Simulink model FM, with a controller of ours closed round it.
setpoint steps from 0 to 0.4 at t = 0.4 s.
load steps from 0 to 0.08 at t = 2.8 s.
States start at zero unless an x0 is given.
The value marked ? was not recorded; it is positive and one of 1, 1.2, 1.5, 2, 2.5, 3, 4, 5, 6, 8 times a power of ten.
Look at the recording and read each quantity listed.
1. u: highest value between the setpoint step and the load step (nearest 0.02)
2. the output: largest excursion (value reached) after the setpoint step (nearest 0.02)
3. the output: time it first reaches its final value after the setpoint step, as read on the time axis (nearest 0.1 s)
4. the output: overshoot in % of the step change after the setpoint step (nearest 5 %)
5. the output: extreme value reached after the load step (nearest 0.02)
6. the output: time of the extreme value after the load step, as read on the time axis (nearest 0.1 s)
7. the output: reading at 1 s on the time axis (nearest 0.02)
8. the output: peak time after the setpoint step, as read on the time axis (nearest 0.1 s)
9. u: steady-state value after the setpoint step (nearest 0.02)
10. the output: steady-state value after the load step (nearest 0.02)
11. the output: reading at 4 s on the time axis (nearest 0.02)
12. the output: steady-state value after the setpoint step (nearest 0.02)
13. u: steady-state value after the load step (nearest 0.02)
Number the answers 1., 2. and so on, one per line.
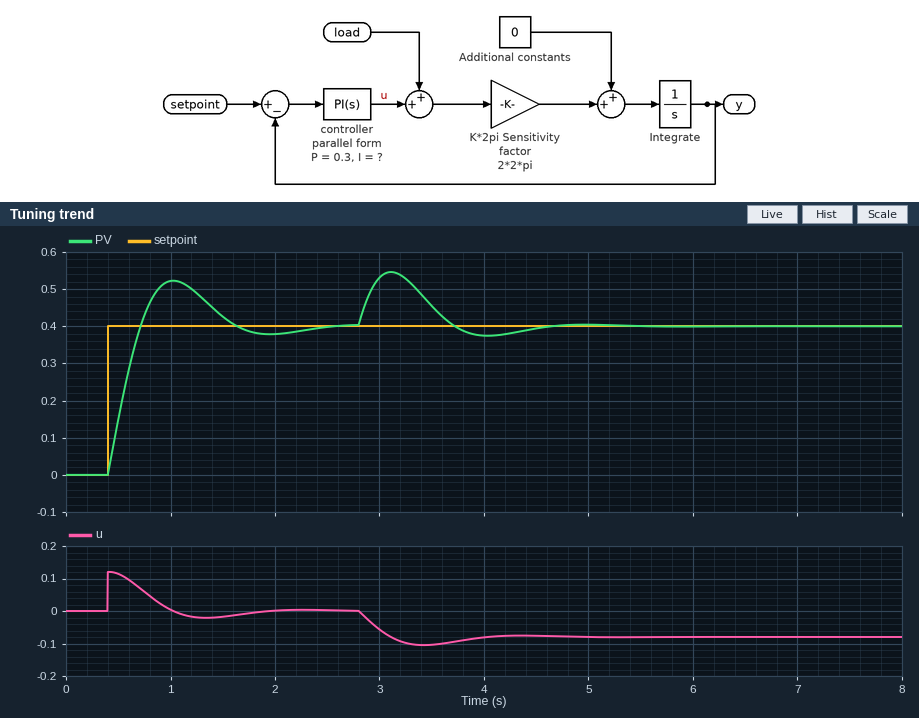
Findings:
1. 0.12
2. 0.52
3. 0.7 s
4. 30 %
5. 0.54
6. 3.1 s
7. 0.52
8. 1.0 s
9. 0.00
10. 0.40
11. 0.38
12. 0.40
13. -0.08
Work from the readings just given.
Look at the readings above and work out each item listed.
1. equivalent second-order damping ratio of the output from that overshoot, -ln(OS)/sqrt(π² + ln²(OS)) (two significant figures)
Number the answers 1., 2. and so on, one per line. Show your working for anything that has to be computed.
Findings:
1. ln(0.3) = -1.204; 1.204 / sqrt(9.870 + 1.450) = 0.36
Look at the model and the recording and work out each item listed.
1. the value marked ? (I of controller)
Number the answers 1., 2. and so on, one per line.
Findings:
1. 1.2
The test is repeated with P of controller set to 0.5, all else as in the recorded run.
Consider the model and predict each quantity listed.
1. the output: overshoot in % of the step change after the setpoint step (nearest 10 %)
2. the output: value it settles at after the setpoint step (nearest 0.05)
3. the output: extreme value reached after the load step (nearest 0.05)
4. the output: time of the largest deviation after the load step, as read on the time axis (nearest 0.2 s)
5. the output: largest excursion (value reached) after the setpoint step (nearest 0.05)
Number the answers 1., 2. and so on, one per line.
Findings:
1. 20 %
2. 0.40
3. 0.50
4. 3.0 s
5. 0.45
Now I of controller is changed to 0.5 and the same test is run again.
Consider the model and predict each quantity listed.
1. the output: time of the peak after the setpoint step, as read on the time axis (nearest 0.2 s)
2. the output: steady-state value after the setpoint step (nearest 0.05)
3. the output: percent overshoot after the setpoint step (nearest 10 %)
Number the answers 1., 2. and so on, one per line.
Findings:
1. 1.2 s
2. 0.40
3. 20 %
